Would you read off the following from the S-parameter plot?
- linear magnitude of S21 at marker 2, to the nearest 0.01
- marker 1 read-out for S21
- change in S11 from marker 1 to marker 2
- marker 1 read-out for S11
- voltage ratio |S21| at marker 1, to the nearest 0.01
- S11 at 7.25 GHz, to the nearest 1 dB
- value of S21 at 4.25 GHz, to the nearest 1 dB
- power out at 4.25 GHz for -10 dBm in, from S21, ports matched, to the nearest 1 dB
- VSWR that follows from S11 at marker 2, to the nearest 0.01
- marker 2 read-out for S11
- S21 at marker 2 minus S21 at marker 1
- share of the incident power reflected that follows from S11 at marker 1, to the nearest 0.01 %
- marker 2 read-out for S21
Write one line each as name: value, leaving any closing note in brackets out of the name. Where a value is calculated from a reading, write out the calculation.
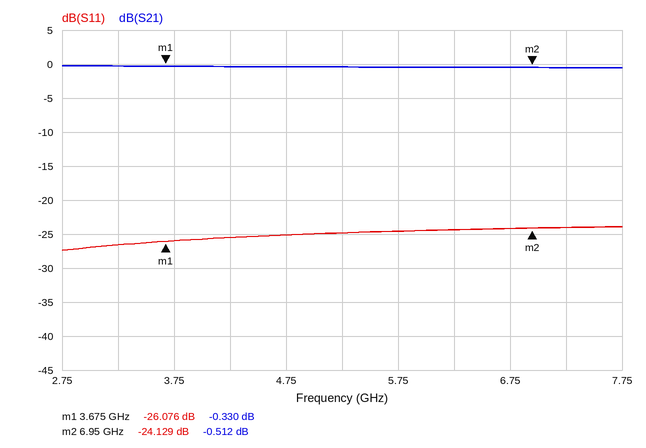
linear magnitude of S21 at marker 2, to the nearest 0.01: 10^(-0.512/20) ≈ 0.94
marker 1 read-out for S21: -0.330 dB
change in S11 from marker 1 to marker 2: -24.129 − (-26.076) = 1.947 dB
marker 1 read-out for S11: -26.076 dB
voltage ratio |S21| at marker 1, to the nearest 0.01: 10^(-0.33/20) ≈ 0.96
S11 at 7.25 GHz, to the nearest 1 dB: -24 dB
value of S21 at 4.25 GHz, to the nearest 1 dB: 0 dB
power out at 4.25 GHz for -10 dBm in, from S21, ports matched, to the nearest 1 dB: -10 dBm + (0 dB) = -10 dBm
VSWR that follows from S11 at marker 2, to the nearest 0.01: (1 + 0.0622)/(1 − 0.0622) ≈ 1.13
marker 2 read-out for S11: -24.129 dB
S21 at marker 2 minus S21 at marker 1: -0.512 − (-0.33) = -0.182 dB
share of the incident power reflected that follows from S11 at marker 1, to the nearest 0.01 %: 10^(-26.076/10) ≈ 0.25 %
marker 2 read-out for S21: -0.512 dB
